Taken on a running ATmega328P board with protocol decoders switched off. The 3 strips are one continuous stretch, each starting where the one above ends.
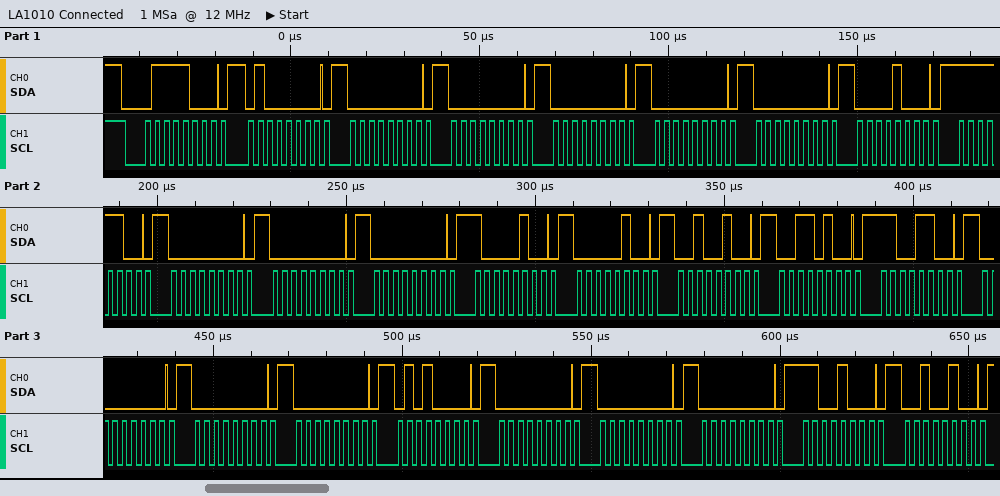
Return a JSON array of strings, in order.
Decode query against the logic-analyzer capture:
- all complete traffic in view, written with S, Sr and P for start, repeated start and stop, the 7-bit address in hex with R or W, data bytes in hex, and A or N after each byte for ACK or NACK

["S 3CW A 40 A 00 A 00 A 00 A 00 A 00 A 08 A FC A 00 A 00 A 00 A 84 A 04 A 24 A 34 A CC A 00 A 00 A 00 A 50 A 00 A 00 A 00 A C8 A 24 A"]
